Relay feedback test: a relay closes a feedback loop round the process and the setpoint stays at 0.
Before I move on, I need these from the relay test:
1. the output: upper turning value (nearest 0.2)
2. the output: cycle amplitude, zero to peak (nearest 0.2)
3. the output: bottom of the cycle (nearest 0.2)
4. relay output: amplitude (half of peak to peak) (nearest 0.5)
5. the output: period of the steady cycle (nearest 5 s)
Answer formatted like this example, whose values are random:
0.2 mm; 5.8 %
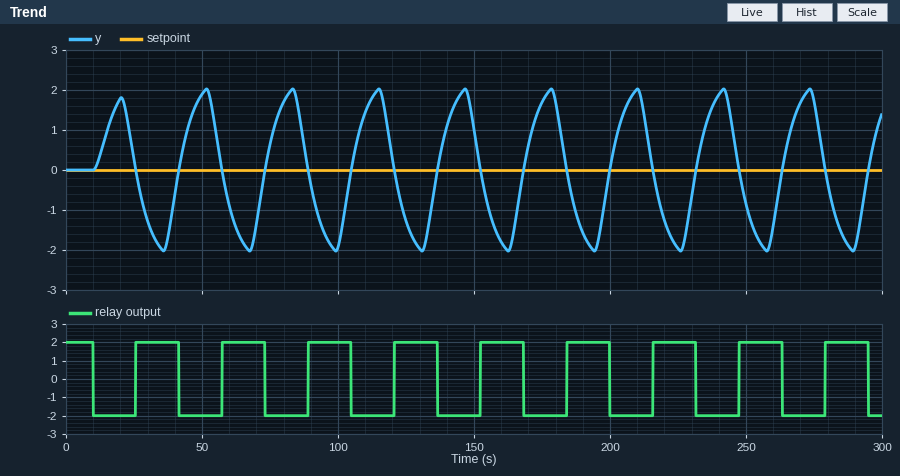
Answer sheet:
2.0; 2.0; -2.0; 2.0; 30 s
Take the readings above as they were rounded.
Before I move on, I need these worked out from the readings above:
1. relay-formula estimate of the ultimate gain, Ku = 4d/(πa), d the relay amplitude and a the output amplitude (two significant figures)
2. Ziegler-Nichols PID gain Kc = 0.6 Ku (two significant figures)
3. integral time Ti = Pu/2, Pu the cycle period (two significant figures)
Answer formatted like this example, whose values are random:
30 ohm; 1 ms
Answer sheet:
1.3; 0.78; 15 s
